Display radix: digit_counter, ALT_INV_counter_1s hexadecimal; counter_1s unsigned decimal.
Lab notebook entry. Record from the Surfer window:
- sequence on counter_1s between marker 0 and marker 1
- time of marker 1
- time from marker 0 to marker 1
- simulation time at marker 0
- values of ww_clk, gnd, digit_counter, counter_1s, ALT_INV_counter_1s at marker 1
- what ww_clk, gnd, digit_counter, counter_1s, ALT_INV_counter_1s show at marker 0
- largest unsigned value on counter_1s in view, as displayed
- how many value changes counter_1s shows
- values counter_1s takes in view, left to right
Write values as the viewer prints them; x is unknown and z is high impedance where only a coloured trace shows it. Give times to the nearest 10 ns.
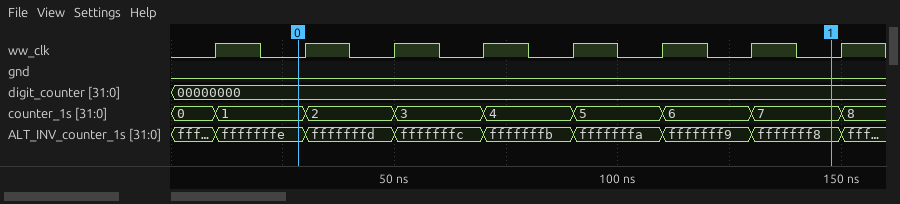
1, 2, 3, 4, 5, 6, 7
150 ns
120 ns
30 ns
ww_clk=0, gnd=0, digit_counter=00000000, counter_1s=7, ALT_INV_counter_1s=fffffff8
ww_clk=0, gnd=0, digit_counter=00000000, counter_1s=1, ALT_INV_counter_1s=fffffffe
8
8
0, 1, 2, 3, 4, 5, 6, 7, 8
